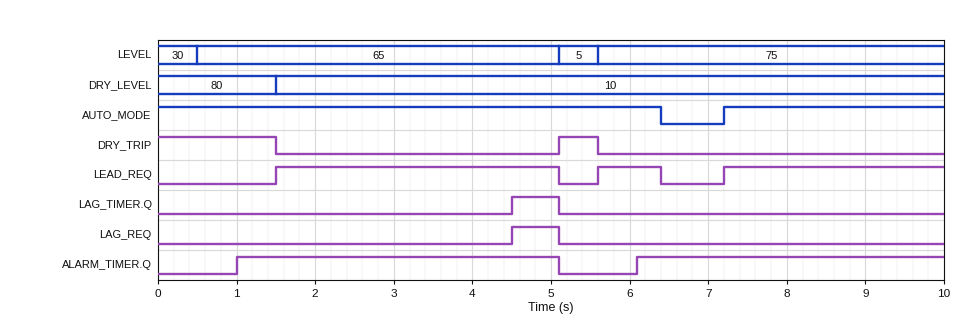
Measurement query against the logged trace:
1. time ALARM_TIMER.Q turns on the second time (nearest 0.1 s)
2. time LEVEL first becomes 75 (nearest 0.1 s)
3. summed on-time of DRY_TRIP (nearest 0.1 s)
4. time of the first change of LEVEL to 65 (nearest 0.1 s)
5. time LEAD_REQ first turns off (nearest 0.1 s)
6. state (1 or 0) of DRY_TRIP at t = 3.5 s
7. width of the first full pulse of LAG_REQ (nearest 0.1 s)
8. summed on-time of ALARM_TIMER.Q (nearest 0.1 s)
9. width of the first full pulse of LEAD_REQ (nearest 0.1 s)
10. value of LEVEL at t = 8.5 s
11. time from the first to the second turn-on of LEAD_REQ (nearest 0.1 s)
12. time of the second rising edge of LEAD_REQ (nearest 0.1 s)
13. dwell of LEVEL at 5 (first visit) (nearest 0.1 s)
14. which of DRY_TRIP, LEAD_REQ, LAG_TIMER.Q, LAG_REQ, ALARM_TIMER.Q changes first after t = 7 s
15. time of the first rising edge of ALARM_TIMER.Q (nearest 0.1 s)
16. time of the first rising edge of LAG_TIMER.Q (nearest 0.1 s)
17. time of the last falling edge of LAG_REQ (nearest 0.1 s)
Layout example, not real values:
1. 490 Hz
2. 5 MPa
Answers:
1. 6.1 s
2. 5.6 s
3. 2.0 s
4. 0.5 s
5. 5.1 s
6. 0
7. 0.6 s
8. 8.0 s
9. 3.6 s
10. 75
11. 4.1 s
12. 5.6 s
13. 0.5 s
14. LEAD_REQ
15. 1.0 s
16. 4.5 s
17. 5.1 s
